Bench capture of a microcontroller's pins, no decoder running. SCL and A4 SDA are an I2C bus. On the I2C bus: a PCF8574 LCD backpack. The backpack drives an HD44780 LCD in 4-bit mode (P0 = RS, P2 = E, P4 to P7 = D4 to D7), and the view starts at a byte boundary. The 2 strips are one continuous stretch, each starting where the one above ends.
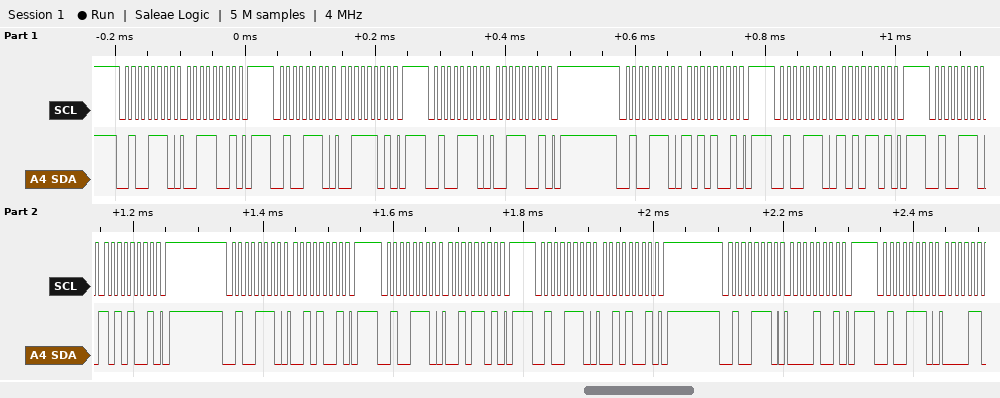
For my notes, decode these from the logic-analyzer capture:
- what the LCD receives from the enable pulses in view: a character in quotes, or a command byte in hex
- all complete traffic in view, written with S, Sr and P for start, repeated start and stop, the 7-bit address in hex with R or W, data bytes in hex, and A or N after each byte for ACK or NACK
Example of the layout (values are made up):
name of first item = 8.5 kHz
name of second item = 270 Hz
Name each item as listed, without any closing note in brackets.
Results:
what the LCD receives from the enable pulses in view: a character in quotes, or a command byte in hex = ':'
all complete traffic in view, written with S, Sr and P for start, repeated start and stop, the 7-bit address in hex with R or W, data bytes in hex, and A or N after each byte for ACK or NACK = S 27W A 39 A P S 27W A 3D A P S 27W A 39 A P S 27W A A9 A P S 27W A AD A P S 27W A A9 A P S 27W A 29 A P S 27W A 2D A P S 27W A 29 A P S 27W A 09 A P S 27W A
